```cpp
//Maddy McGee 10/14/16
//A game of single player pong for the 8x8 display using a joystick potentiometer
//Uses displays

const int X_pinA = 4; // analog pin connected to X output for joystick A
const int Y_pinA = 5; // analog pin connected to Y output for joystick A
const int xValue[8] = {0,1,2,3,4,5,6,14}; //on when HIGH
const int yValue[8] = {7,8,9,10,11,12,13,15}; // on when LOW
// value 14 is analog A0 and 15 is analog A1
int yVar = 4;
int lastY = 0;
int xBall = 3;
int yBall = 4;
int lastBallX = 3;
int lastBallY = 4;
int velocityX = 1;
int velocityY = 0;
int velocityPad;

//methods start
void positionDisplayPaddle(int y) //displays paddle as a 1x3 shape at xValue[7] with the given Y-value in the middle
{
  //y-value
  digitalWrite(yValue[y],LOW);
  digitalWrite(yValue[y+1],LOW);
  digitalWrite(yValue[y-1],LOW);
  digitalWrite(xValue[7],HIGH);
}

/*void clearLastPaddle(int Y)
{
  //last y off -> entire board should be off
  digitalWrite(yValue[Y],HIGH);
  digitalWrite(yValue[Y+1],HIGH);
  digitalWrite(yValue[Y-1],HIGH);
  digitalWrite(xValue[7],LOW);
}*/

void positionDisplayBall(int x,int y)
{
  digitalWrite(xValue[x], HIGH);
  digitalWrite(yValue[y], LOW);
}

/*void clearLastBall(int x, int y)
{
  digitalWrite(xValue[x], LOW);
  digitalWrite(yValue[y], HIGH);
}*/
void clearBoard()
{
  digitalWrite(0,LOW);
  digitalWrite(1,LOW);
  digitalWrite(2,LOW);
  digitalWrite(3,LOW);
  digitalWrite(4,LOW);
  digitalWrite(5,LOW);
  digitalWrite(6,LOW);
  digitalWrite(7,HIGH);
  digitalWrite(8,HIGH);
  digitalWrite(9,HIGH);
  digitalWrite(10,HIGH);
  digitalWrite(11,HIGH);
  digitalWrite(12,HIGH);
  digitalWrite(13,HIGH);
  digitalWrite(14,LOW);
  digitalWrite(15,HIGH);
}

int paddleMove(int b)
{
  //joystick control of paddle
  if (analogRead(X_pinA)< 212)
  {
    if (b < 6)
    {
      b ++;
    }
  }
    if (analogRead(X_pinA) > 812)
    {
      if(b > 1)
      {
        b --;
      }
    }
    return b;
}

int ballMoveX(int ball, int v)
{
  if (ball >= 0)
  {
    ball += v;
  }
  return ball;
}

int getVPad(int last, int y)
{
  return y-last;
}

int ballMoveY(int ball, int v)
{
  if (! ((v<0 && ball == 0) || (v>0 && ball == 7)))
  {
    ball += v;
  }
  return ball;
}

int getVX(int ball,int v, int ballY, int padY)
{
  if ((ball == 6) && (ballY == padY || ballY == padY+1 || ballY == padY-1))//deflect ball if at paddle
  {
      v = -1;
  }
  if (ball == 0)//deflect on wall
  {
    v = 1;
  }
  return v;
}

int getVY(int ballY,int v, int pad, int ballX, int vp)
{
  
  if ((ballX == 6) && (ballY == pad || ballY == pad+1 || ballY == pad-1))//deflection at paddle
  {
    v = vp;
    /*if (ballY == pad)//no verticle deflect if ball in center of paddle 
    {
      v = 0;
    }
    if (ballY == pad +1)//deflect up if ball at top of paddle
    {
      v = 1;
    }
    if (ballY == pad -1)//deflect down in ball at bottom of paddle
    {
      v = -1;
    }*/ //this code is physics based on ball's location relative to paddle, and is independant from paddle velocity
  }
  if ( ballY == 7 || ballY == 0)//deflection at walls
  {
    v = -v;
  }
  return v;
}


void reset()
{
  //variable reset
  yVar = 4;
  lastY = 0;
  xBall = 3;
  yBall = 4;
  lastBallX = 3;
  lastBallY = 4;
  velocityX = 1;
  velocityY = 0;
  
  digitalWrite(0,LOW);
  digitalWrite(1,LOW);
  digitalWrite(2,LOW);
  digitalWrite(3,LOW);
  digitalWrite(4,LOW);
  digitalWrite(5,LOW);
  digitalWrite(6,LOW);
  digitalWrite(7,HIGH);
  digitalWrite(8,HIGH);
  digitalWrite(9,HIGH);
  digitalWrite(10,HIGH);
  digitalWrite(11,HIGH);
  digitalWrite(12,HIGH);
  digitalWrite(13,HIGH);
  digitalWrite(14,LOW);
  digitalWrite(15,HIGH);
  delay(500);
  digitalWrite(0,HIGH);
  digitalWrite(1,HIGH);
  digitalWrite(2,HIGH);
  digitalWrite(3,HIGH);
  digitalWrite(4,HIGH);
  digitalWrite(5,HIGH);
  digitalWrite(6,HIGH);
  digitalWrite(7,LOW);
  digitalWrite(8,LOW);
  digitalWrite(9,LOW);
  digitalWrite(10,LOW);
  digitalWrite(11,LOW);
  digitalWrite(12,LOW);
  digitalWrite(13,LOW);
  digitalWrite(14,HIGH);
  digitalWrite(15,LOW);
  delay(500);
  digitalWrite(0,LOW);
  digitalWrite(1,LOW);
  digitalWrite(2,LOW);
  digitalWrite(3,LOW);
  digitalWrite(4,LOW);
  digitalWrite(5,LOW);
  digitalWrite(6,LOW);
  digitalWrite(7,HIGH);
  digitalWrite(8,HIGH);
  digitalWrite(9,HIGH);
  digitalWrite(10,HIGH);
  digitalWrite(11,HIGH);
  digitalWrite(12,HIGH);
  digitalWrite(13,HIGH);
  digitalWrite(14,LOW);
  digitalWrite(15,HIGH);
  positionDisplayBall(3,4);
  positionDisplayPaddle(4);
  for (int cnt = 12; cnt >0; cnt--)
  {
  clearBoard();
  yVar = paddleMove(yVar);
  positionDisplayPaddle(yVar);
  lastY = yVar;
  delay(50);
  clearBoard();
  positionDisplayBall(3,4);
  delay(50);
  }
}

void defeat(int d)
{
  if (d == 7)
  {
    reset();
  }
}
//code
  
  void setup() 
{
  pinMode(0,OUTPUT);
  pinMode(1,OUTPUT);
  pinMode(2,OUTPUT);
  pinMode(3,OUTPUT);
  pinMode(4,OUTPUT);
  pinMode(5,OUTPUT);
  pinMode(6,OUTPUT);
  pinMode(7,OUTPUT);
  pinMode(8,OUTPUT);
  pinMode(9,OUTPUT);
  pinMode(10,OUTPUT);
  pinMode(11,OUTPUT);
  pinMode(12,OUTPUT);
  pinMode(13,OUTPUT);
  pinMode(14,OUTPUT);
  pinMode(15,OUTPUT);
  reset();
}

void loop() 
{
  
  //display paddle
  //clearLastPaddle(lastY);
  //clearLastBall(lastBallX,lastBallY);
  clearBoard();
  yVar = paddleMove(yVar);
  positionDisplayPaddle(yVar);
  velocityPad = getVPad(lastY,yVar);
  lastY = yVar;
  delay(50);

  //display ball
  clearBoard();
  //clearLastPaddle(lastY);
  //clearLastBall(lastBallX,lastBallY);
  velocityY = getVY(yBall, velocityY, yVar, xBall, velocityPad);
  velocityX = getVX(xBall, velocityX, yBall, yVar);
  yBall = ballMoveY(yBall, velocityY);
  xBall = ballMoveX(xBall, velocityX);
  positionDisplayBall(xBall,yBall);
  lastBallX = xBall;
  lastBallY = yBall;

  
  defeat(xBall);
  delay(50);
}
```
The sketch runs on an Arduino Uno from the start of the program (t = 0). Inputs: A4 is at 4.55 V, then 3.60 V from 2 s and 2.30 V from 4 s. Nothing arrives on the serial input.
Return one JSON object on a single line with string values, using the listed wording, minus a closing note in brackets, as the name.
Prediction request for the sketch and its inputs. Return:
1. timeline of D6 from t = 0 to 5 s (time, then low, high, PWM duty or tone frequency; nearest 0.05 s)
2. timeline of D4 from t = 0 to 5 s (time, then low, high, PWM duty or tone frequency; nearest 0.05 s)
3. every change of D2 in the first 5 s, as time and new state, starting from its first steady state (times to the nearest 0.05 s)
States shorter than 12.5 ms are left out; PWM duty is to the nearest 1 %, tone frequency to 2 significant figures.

{"timeline of D6 from t = 0 to 5 s": "0 s low; 0.5 s high; 1 s low; 2.45 s high; 2.5 s low; 3.05 s high; 3.55 s low", "timeline of D4 from t = 0 to 5 s": "0 s low; 0.5 s high; 1 s low; 2.25 s high; 2.3 s low; 3.05 s high; 3.55 s low; 4.85 s high; 4.9 s low", "every change of D2 in the first 5 s, as time and new state, starting from its first steady state": "0 s low; 0.5 s high; 1 s low; 3.05 s high; 3.55 s low"}
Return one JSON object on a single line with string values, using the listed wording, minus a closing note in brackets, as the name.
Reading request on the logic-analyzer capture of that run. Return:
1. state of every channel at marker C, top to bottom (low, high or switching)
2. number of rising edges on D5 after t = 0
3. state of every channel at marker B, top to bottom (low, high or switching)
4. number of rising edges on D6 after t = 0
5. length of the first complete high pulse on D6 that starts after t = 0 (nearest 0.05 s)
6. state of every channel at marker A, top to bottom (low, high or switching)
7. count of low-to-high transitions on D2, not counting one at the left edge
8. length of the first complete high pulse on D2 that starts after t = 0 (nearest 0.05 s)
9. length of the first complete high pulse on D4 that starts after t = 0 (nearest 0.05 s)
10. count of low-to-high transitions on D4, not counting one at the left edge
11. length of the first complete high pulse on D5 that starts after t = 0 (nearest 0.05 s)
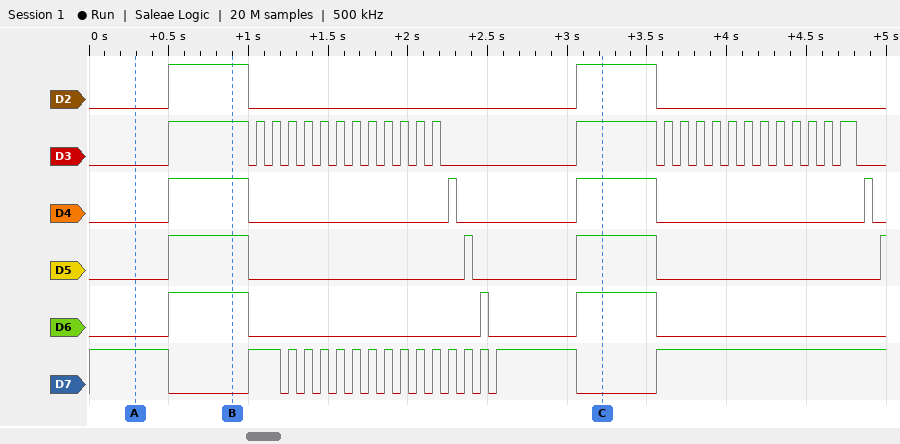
{"state of every channel at marker C, top to bottom": "D2 high, D3 high, D4 high, D5 high, D6 high, D7 low", "number of rising edges on D5 after t = 0": "4", "state of every channel at marker B, top to bottom": "D2 high, D3 high, D4 high, D5 high, D6 high, D7 low", "number of rising edges on D6 after t = 0": "3", "length of the first complete high pulse on D6 that starts after t = 0": "0.50 s", "state of every channel at marker A, top to bottom": "D2 low, D3 low, D4 low, D5 low, D6 low, D7 high", "count of low-to-high transitions on D2, not counting one at the left edge": "2", "length of the first complete high pulse on D2 that starts after t = 0": "0.50 s", "length of the first complete high pulse on D4 that starts after t = 0": "0.50 s", "count of low-to-high transitions on D4, not counting one at the left edge": "4", "length of the first complete high pulse on D5 that starts after t = 0": "0.50 s"}
